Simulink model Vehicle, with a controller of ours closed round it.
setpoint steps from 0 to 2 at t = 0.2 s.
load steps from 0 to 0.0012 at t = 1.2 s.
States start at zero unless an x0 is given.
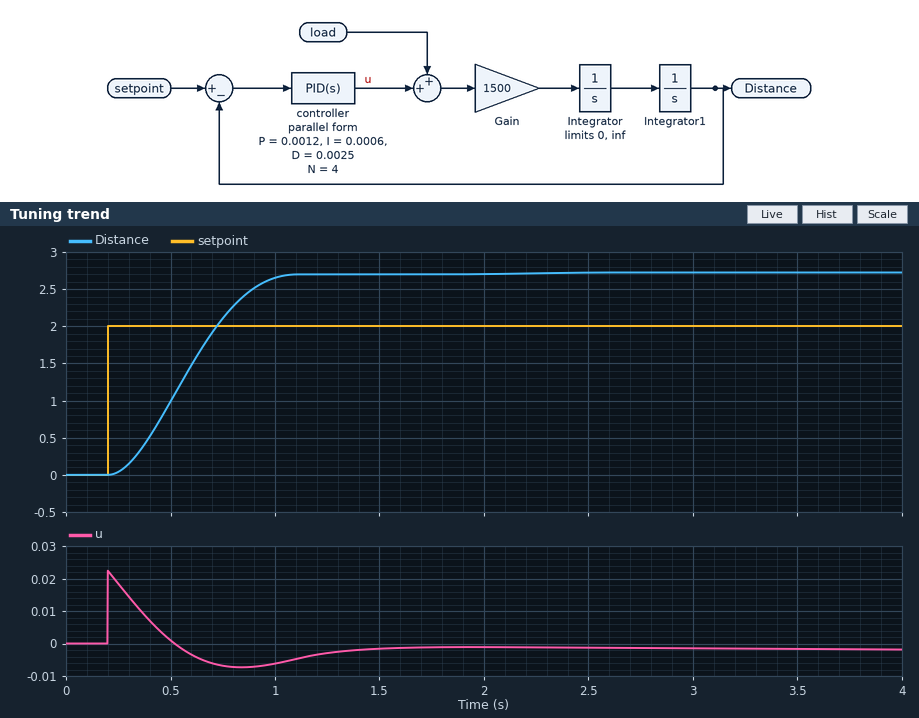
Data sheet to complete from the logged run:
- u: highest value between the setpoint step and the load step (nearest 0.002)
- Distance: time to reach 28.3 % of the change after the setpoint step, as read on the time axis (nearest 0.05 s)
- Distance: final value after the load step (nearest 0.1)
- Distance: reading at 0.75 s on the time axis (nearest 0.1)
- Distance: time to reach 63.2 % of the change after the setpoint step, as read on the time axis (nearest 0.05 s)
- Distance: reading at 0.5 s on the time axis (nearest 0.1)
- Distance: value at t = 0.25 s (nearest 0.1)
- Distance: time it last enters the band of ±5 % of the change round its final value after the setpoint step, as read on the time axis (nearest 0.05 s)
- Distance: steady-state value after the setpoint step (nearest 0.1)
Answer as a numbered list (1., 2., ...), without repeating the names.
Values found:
1. 0.022
2. 0.45 s
3. 2.7
4. 2.1
5. 0.65 s
6. 1.0
7. 0.0
8. 0.95 s
9. 2.7
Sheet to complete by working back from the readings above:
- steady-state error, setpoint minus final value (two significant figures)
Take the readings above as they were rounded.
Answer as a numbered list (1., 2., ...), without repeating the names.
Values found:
1. -0.70
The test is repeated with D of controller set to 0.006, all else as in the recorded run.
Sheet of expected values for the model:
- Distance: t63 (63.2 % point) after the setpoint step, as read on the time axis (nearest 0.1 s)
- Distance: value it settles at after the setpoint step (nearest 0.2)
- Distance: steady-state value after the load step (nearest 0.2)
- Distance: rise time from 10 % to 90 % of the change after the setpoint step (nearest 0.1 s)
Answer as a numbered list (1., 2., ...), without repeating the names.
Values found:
1. 0.5 s
2. 2.8
3. 2.8
4. 0.3 s
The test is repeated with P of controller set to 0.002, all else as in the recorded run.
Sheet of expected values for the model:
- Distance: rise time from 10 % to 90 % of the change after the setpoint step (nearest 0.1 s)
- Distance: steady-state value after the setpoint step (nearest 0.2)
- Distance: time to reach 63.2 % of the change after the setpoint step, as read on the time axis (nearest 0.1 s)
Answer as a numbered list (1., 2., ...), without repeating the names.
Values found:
1. 0.5 s
2. 2.8
3. 0.6 s
